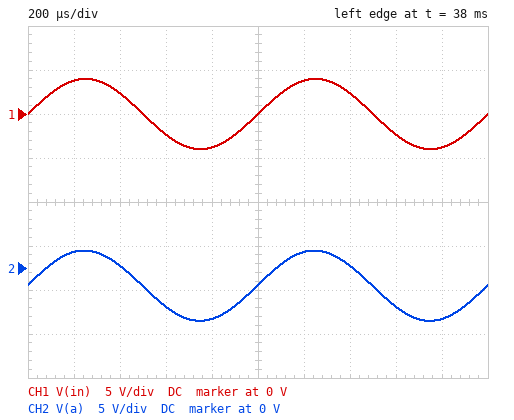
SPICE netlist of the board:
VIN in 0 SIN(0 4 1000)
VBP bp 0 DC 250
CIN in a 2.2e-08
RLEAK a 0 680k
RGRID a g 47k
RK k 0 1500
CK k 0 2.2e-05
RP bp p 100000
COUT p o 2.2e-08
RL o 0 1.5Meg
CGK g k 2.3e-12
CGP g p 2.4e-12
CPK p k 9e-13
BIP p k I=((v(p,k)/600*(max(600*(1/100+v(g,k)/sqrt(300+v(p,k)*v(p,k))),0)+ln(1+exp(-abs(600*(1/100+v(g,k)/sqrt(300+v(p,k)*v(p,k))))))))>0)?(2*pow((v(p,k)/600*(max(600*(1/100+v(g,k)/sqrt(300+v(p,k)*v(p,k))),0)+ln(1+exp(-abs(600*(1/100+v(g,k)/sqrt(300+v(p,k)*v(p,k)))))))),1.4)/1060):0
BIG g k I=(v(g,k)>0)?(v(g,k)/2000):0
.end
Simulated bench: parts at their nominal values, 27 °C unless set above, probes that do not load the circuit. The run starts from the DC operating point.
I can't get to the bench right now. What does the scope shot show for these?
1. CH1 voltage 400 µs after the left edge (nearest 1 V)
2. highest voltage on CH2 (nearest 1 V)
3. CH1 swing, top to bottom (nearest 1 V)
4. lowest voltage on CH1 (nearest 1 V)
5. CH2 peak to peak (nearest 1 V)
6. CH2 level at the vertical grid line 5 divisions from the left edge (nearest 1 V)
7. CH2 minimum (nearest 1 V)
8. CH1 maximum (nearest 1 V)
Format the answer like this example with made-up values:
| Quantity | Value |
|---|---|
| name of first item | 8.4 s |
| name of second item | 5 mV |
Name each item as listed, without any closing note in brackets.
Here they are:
| Quantity | Value |
|---|---|
| CH1 voltage 400 µs after the left edge | 2 V |
| highest voltage on CH2 | 2 V |
| CH1 swing, top to bottom | 8 V |
| lowest voltage on CH1 | -4 V |
| CH2 peak to peak | 8 V |
| CH2 level at the vertical grid line 5 divisions from the left edge | -2 V |
| CH2 minimum | -6 V |
| CH1 maximum | 4 V |
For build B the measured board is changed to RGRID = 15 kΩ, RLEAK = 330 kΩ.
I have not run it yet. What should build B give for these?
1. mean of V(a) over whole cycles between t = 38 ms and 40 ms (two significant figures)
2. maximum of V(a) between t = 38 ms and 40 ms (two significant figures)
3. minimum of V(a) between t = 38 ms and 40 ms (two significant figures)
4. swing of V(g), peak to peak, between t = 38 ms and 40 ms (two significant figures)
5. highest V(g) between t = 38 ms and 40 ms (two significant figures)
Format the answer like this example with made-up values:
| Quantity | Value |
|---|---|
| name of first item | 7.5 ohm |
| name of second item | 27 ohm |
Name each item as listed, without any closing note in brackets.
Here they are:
| Quantity | Value |
|---|---|
| mean of V(a) over whole cycles between t = 38 ms and 40 ms | -2.2 V |
| maximum of V(a) between t = 38 ms and 40 ms | 1.8 V |
| minimum of V(a) between t = 38 ms and 40 ms | -6.2 V |
| swing of V(g), peak to peak, between t = 38 ms and 40 ms | 7.2 V |
| highest V(g) between t = 38 ms and 40 ms | 1.1 V |
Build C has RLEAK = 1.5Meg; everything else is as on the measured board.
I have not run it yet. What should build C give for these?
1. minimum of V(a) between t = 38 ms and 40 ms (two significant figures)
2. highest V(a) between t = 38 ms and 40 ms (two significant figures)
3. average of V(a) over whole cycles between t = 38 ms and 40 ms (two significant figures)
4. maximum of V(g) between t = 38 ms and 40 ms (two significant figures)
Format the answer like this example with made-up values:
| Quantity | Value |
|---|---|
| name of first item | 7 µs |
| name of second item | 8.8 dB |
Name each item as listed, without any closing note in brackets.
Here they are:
| Quantity | Value |
|---|---|
| minimum of V(a) between t = 38 ms and 40 ms | -6.4 V |
| highest V(a) between t = 38 ms and 40 ms | 1.6 V |
| average of V(a) over whole cycles between t = 38 ms and 40 ms | -2.4 V |
| maximum of V(g) between t = 38 ms and 40 ms | 980 mV |
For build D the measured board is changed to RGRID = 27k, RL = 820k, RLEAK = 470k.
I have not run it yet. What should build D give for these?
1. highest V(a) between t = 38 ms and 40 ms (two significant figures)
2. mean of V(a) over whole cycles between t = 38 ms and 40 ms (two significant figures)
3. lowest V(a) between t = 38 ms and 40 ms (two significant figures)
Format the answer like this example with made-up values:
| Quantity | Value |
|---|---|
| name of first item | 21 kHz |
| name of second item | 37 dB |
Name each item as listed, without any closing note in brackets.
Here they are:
| Quantity | Value |
|---|---|
| highest V(a) between t = 38 ms and 40 ms | 1.9 V |
| mean of V(a) over whole cycles between t = 38 ms and 40 ms | -2.1 V |
| lowest V(a) between t = 38 ms and 40 ms | -6.1 V |
